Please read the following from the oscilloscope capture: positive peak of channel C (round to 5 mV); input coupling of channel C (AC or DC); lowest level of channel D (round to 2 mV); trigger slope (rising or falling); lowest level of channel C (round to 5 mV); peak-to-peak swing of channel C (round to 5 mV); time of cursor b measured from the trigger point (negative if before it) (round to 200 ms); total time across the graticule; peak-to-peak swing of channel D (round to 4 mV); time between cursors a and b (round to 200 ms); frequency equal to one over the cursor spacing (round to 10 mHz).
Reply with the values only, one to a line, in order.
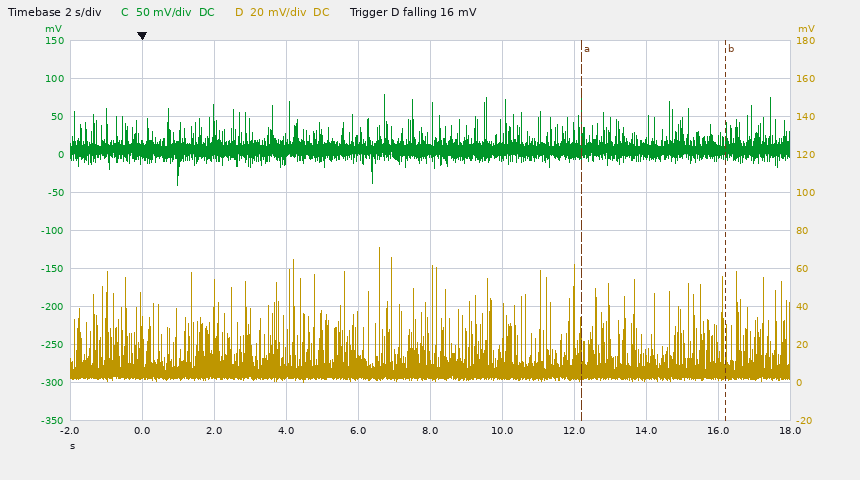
80 mV
DC
0 mV
falling
-40 mV
120 mV
+16.2 s
20 s
72 mV
4.0 s
250 mHz
